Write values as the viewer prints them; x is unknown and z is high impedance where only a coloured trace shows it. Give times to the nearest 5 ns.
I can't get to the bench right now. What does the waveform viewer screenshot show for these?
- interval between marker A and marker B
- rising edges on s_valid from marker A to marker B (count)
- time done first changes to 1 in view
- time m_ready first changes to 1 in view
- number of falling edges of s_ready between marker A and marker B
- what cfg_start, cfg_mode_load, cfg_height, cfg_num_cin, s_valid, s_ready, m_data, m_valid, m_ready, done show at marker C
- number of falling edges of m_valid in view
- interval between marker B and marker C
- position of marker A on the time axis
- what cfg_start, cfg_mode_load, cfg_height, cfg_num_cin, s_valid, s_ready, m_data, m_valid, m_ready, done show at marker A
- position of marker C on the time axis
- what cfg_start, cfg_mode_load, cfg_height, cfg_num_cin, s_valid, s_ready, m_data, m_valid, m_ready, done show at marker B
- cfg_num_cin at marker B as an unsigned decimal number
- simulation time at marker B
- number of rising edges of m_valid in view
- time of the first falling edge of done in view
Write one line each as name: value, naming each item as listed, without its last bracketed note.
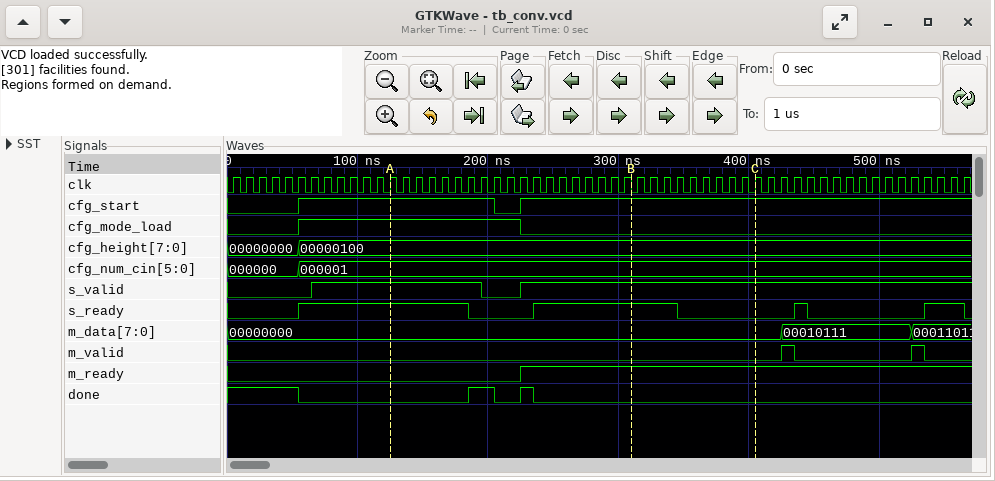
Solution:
interval between marker A and marker B: 185 ns
rising edges on s_valid from marker A to marker B: 1
time done first changes to 1 in view: 185 ns
time m_ready first changes to 1 in view: 225 ns
number of falling edges of s_ready between marker A and marker B: 1
what cfg_start, cfg_mode_load, cfg_height, cfg_num_cin, s_valid, s_ready, m_data, m_valid, m_ready, done show at marker C: cfg_start=1, cfg_mode_load=0, cfg_height=00000100, cfg_num_cin=000001, s_valid=1, s_ready=0, m_data=00000000, m_valid=0, m_ready=1, done=0
number of falling edges of m_valid in view: 2
interval between marker B and marker C: 95 ns
position of marker A on the time axis: 125 ns
what cfg_start, cfg_mode_load, cfg_height, cfg_num_cin, s_valid, s_ready, m_data, m_valid, m_ready, done show at marker A: cfg_start=1, cfg_mode_load=1, cfg_height=00000100, cfg_num_cin=000001, s_valid=1, s_ready=1, m_data=00000000, m_valid=0, m_ready=0, done=0
position of marker C on the time axis: 405 ns
what cfg_start, cfg_mode_load, cfg_height, cfg_num_cin, s_valid, s_ready, m_data, m_valid, m_ready, done show at marker B: cfg_start=1, cfg_mode_load=0, cfg_height=00000100, cfg_num_cin=000001, s_valid=1, s_ready=1, m_data=00000000, m_valid=0, m_ready=1, done=0
cfg_num_cin at marker B as an unsigned decimal number: 1
simulation time at marker B: 310 ns
number of rising edges of m_valid in view: 2
time of the first falling edge of done in view: 55 ns
